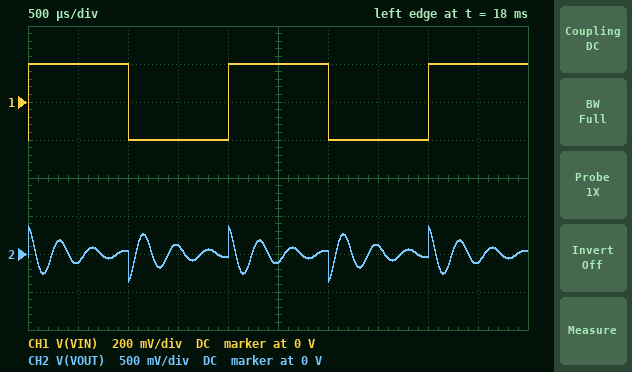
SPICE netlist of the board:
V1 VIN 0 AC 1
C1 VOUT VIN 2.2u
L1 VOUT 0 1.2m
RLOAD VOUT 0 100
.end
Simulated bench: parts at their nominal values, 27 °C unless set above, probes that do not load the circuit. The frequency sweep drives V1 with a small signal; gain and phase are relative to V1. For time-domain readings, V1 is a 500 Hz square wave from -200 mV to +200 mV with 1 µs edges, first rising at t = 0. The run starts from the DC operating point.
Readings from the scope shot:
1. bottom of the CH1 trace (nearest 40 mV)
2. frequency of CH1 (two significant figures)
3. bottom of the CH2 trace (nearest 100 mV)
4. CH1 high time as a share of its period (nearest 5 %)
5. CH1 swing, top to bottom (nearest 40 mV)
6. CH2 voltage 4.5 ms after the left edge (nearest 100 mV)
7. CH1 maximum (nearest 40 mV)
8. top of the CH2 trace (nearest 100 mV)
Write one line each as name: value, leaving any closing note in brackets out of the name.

bottom of the CH1 trace: -200 mV
frequency of CH1: 500 Hz
bottom of the CH2 trace: -400 mV
CH1 high time as a share of its period: 50 %
CH1 swing, top to bottom: 400 mV
CH2 voltage 4.5 ms after the left edge: -100 mV
CH1 maximum: 200 mV
top of the CH2 trace: 400 mV
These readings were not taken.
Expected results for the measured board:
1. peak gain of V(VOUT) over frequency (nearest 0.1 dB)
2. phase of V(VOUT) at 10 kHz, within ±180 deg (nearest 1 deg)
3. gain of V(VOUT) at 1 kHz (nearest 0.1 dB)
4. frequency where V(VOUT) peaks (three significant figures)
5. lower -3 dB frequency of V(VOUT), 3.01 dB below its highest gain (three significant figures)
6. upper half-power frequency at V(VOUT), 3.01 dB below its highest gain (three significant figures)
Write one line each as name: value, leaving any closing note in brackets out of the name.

peak gain of V(VOUT) over frequency: 12.7 dB
phase of V(VOUT) at 10 kHz, within ±180 deg: 5 deg
gain of V(VOUT) at 1 kHz: -18.7 dB
frequency where V(VOUT) peaks: 3.14 kHz
lower -3 dB frequency of V(VOUT), 3.01 dB below its highest gain: 2.82 kHz
upper half-power frequency at V(VOUT), 3.01 dB below its highest gain: 3.60 kHz
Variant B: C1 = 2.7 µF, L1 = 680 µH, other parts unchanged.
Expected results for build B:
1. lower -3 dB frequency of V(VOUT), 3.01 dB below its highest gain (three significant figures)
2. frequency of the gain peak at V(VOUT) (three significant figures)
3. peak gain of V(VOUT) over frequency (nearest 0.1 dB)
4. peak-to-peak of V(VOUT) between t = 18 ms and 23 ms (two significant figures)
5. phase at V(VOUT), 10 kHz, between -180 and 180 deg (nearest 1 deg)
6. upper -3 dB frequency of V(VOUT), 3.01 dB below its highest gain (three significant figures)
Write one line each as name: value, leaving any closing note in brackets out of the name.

lower -3 dB frequency of V(VOUT), 3.01 dB below its highest gain: 3.47 kHz
frequency of the gain peak at V(VOUT): 3.74 kHz
peak gain of V(VOUT) over frequency: 16.0 dB
peak-to-peak of V(VOUT) between t = 18 ms and 23 ms: 810 mV
phase at V(VOUT), 10 kHz, between -180 and 180 deg: 4 deg
upper -3 dB frequency of V(VOUT), 3.01 dB below its highest gain: 4.08 kHz
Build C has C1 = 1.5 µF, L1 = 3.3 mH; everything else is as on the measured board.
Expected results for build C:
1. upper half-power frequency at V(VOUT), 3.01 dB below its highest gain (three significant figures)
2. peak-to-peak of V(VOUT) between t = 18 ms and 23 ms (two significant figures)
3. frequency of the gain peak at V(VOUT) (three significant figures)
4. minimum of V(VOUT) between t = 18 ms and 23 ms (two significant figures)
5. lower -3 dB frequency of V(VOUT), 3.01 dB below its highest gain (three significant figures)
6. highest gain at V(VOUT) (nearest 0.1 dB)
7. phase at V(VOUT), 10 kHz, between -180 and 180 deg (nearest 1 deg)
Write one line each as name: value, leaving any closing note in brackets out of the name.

upper half-power frequency at V(VOUT), 3.01 dB below its highest gain: 3.43 kHz
peak-to-peak of V(VOUT) between t = 18 ms and 23 ms: 790 mV
frequency of the gain peak at V(VOUT): 2.40 kHz
minimum of V(VOUT) between t = 18 ms and 23 ms: -400 mV
lower -3 dB frequency of V(VOUT), 3.01 dB below its highest gain: 1.95 kHz
highest gain at V(VOUT): 6.8 dB
phase at V(VOUT), 10 kHz, between -180 and 180 deg: 6 deg
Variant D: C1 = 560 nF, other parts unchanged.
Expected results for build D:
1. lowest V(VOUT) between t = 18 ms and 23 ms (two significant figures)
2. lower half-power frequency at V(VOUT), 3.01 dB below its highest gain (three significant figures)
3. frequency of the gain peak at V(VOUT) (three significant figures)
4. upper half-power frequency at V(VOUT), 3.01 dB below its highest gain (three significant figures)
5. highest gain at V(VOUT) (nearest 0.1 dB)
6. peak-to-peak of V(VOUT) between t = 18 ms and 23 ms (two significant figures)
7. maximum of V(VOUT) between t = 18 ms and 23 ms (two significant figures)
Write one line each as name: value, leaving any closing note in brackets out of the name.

lowest V(VOUT) between t = 18 ms and 23 ms: -400 mV
lower half-power frequency at V(VOUT), 3.01 dB below its highest gain: 5.30 kHz
frequency of the gain peak at V(VOUT): 6.50 kHz
upper half-power frequency at V(VOUT), 3.01 dB below its highest gain: 9.23 kHz
highest gain at V(VOUT): 6.9 dB
peak-to-peak of V(VOUT) between t = 18 ms and 23 ms: 790 mV
maximum of V(VOUT) between t = 18 ms and 23 ms: 400 mV
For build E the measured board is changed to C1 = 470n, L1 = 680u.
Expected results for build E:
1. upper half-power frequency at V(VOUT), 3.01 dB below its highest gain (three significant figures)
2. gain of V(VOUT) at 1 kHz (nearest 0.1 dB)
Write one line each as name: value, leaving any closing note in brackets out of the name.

upper half-power frequency at V(VOUT), 3.01 dB below its highest gain: 12.0 kHz
gain of V(VOUT) at 1 kHz: -37.9 dB
